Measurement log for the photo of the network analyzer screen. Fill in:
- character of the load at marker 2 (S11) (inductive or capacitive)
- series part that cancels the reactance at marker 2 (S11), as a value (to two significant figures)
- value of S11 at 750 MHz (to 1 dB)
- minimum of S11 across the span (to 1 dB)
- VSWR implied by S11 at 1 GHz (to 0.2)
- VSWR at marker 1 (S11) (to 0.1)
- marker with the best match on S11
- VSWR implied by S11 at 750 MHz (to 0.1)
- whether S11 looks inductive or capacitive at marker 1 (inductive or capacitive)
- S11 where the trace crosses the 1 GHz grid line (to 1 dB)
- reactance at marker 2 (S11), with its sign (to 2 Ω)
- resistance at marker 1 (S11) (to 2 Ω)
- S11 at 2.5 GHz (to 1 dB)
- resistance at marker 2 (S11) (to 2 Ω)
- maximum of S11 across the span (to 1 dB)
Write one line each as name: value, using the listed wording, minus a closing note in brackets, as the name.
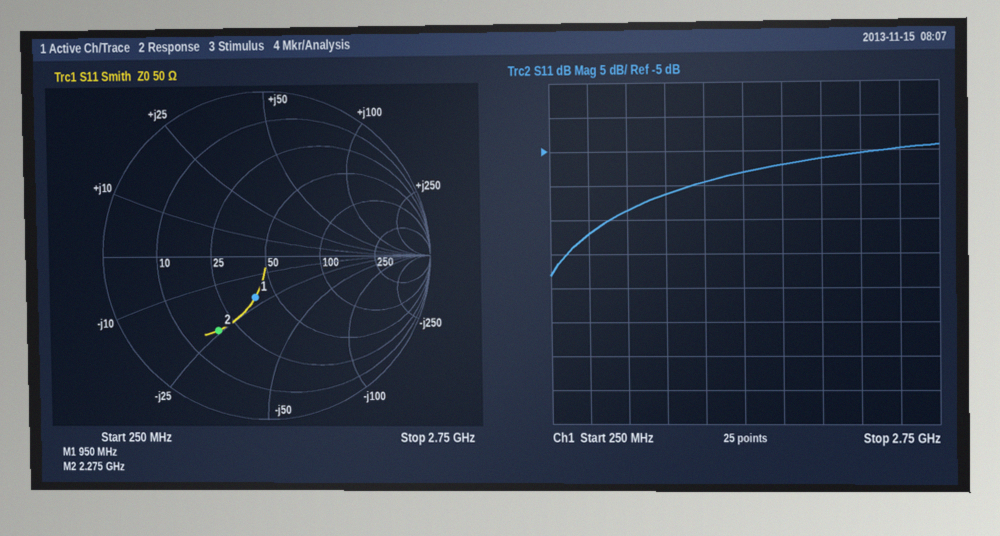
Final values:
character of the load at marker 2 (S11): capacitive
series part that cancels the reactance at marker 2 (S11), as a value: 1.7 nH
value of S11 at 750 MHz: -14 dB
minimum of S11 across the span: -23 dB
VSWR implied by S11 at 1 GHz: 1.8
VSWR at marker 1 (S11): 1.7
marker with the best match on S11: marker 1
VSWR implied by S11 at 750 MHz: 1.5
whether S11 looks inductive or capacitive at marker 1: capacitive
S11 where the trace crosses the 1 GHz grid line: -11 dB
reactance at marker 2 (S11), with its sign: -24 Ω
resistance at marker 1 (S11): 38 Ω
S11 at 2.5 GHz: -5 dB
resistance at marker 2 (S11): 18 Ω
maximum of S11 across the span: -4 dB
